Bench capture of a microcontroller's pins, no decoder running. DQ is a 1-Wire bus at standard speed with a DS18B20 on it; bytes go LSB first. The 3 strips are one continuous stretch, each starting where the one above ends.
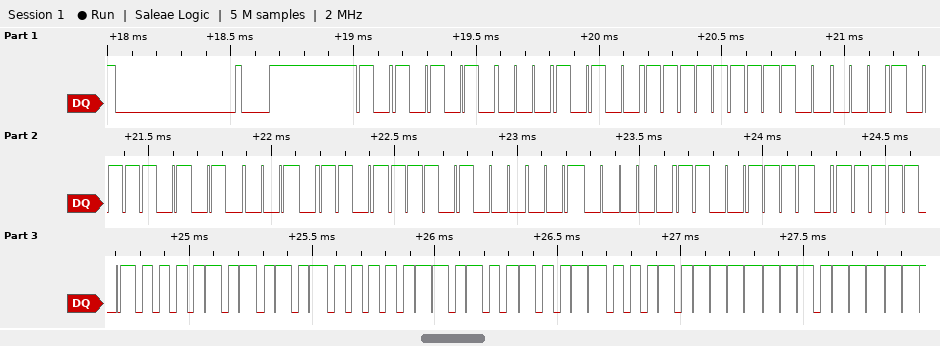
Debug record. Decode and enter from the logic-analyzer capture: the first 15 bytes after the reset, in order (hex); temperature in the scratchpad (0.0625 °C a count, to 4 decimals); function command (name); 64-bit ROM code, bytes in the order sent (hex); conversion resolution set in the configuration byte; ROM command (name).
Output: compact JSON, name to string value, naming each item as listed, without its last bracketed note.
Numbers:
{"the first 15 bytes after the reset, in order": "55 28 FF 41 57 B4 17 04 F3 BE 50 05 4B 46 7F", "temperature in the scratchpad": "85.0000 °C", "function command": "Read Scratchpad", "64-bit ROM code, bytes in the order sent": "28 FF 41 57 B4 17 04 F3", "conversion resolution set in the configuration byte": "12 bits", "ROM command": "Match ROM"}
